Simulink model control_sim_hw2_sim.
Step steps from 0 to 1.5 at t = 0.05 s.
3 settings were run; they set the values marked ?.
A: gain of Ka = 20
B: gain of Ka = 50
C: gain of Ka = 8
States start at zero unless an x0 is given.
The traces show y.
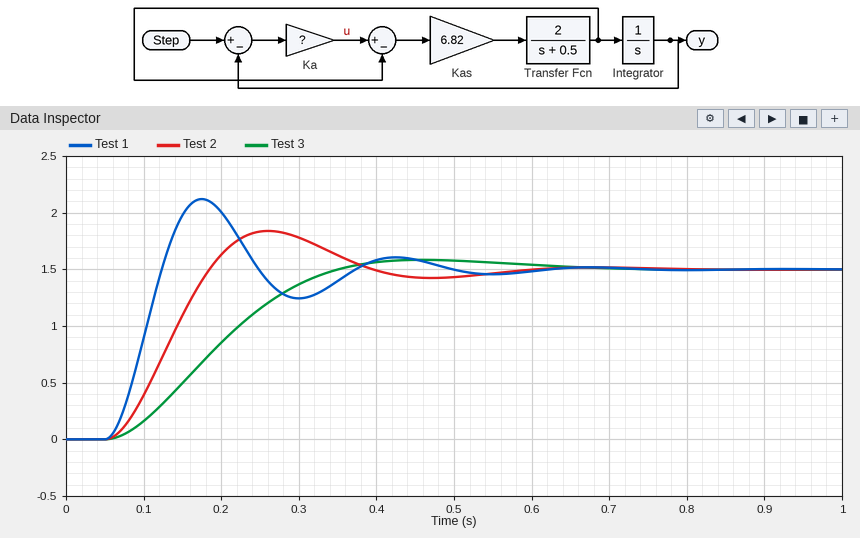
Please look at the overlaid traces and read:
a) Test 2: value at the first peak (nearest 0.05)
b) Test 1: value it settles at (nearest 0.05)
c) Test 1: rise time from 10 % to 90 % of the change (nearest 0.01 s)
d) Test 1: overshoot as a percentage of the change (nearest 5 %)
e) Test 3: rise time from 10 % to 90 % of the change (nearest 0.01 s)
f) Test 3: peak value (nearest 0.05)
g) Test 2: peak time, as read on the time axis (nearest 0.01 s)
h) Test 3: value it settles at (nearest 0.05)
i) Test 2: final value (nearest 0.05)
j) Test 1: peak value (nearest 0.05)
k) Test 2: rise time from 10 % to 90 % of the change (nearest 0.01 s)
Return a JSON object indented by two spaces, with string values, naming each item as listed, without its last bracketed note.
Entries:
{
  "Test 2: value at the first peak": "1.85",
  "Test 1: value it settles at": "1.50",
  "Test 1: rise time from 10 % to 90 % of the change": "0.05 s",
  "Test 1: overshoot as a percentage of the change": "40 %",
  "Test 3: rise time from 10 % to 90 % of the change": "0.20 s",
  "Test 3: peak value": "1.60",
  "Test 2: peak time, as read on the time axis": "0.26 s",
  "Test 3: value it settles at": "1.50",
  "Test 2: final value": "1.50",
  "Test 1: peak value": "2.10",
  "Test 2: rise time from 10 % to 90 % of the change": "0.09 s"
}
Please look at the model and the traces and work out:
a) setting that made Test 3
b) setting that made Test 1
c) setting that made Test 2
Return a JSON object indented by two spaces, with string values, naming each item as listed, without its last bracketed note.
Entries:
{
  "setting that made Test 3": "C",
  "setting that made Test 1": "B",
  "setting that made Test 2": "A"
}
